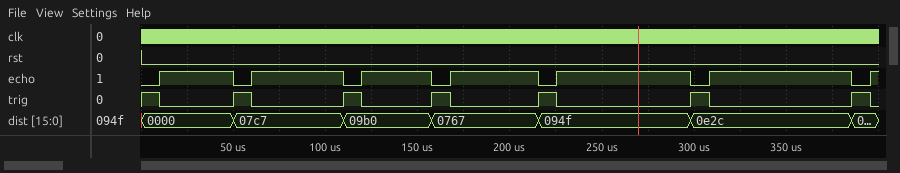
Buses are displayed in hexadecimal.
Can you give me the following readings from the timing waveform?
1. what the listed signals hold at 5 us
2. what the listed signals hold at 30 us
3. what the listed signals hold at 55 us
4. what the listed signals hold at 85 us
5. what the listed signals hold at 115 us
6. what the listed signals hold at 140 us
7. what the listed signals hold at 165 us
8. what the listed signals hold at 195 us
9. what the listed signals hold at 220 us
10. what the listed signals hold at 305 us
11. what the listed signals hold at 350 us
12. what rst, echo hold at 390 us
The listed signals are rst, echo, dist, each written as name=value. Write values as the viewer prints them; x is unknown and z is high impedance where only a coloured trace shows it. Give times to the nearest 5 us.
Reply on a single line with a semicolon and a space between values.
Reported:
rst=0, echo=0, dist=0000; rst=0, echo=1, dist=0000; rst=0, echo=0, dist=07c7; rst=0, echo=1, dist=07c7; rst=0, echo=0, dist=09b0; rst=0, echo=1, dist=09b0; rst=0, echo=0, dist=0767; rst=0, echo=1, dist=0767; rst=0, echo=0, dist=094f; rst=0, echo=0, dist=0e2c; rst=0, echo=1, dist=0e2c; rst=0, echo=0
